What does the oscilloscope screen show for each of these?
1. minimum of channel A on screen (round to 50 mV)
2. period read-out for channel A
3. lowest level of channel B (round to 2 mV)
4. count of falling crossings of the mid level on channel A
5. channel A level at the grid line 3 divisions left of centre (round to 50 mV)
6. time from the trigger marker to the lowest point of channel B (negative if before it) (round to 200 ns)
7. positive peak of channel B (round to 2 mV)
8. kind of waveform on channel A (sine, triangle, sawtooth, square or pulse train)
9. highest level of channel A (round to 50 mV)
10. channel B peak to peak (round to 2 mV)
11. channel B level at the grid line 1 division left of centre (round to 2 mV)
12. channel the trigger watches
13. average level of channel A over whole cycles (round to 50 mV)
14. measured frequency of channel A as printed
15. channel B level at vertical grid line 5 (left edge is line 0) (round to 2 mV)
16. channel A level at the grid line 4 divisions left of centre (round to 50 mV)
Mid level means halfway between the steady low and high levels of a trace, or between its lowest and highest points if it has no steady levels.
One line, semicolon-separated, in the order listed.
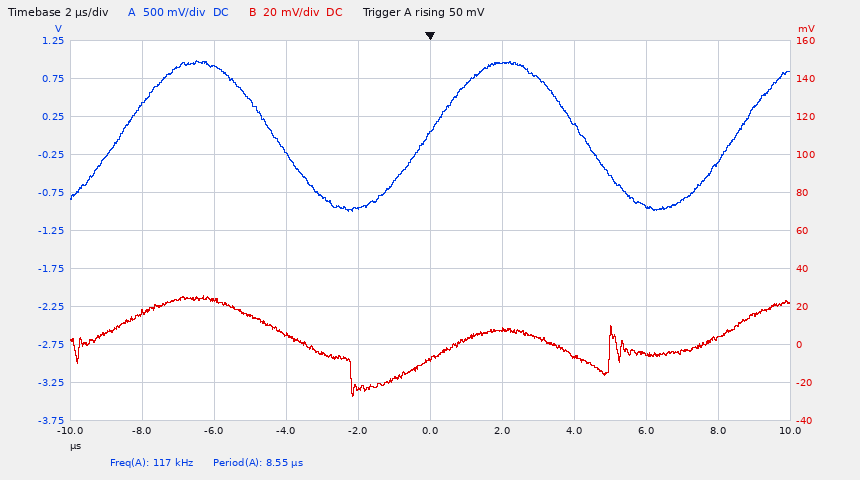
-1.00 V; 8.55 µs; -28 mV; 2; 900 mV; -2.2 µs; 26 mV; sine; 1.00 V; 54 mV; -22 mV; channel A; 0 mV; 117 kHz; -8 mV; 400 mV
